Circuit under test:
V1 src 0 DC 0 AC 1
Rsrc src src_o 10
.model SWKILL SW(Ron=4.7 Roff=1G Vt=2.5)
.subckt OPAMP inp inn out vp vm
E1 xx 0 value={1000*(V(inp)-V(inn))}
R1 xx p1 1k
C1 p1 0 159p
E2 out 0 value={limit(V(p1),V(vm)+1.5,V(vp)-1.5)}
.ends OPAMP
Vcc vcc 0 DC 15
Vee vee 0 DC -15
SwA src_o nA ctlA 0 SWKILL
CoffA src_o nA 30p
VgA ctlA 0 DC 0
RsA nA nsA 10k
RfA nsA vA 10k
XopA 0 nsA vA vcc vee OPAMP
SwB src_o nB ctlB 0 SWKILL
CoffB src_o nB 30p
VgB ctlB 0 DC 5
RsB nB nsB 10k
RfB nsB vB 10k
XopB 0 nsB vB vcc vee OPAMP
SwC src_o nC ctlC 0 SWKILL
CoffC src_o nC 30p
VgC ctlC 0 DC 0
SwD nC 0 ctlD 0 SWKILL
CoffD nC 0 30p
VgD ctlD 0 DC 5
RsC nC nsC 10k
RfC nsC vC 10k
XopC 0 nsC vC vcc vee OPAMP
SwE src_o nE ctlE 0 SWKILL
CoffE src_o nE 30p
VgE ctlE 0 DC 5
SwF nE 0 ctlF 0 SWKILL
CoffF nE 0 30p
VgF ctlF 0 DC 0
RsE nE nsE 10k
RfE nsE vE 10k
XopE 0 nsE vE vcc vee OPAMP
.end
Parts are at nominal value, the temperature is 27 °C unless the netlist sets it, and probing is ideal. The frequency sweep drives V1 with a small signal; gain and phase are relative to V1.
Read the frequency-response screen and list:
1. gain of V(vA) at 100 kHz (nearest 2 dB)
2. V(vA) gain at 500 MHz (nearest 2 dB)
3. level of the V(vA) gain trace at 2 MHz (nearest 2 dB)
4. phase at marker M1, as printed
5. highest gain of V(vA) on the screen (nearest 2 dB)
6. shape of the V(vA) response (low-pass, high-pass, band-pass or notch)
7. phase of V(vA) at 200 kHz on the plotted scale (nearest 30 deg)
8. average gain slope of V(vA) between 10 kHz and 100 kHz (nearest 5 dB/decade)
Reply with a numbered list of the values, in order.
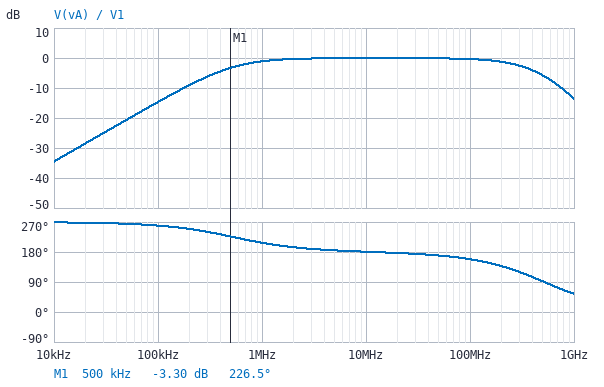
1. -14 dB
2. -6 dB
3. 0 dB
4. 226.5 deg
5. 0 dB
6. band-pass
7. 240 deg
8. 20 dB/decade
